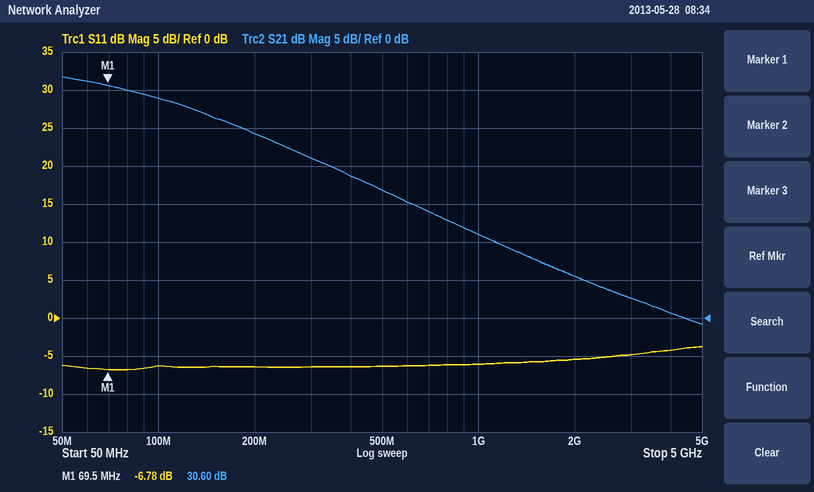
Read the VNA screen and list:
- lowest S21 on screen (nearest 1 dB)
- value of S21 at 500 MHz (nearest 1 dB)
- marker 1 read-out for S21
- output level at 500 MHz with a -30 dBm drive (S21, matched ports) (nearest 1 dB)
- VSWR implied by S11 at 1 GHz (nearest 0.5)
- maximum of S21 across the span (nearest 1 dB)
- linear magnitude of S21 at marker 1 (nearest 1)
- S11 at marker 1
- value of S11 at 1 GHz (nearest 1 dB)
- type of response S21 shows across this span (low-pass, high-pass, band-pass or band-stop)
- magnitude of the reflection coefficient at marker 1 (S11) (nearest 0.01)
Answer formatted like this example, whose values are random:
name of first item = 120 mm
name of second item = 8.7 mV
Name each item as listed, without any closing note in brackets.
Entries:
lowest S21 on screen = -1 dB
value of S21 at 500 MHz = 17 dB
marker 1 read-out for S21 = 30.60 dB
output level at 500 MHz with a -30 dBm drive (S21, matched ports) = -13 dBm
VSWR implied by S11 at 1 GHz = 3.0
maximum of S21 across the span = 32 dB
linear magnitude of S21 at marker 1 = 34
S11 at marker 1 = -6.78 dB
value of S11 at 1 GHz = -6 dB
type of response S21 shows across this span = low-pass
magnitude of the reflection coefficient at marker 1 (S11) = 0.46
